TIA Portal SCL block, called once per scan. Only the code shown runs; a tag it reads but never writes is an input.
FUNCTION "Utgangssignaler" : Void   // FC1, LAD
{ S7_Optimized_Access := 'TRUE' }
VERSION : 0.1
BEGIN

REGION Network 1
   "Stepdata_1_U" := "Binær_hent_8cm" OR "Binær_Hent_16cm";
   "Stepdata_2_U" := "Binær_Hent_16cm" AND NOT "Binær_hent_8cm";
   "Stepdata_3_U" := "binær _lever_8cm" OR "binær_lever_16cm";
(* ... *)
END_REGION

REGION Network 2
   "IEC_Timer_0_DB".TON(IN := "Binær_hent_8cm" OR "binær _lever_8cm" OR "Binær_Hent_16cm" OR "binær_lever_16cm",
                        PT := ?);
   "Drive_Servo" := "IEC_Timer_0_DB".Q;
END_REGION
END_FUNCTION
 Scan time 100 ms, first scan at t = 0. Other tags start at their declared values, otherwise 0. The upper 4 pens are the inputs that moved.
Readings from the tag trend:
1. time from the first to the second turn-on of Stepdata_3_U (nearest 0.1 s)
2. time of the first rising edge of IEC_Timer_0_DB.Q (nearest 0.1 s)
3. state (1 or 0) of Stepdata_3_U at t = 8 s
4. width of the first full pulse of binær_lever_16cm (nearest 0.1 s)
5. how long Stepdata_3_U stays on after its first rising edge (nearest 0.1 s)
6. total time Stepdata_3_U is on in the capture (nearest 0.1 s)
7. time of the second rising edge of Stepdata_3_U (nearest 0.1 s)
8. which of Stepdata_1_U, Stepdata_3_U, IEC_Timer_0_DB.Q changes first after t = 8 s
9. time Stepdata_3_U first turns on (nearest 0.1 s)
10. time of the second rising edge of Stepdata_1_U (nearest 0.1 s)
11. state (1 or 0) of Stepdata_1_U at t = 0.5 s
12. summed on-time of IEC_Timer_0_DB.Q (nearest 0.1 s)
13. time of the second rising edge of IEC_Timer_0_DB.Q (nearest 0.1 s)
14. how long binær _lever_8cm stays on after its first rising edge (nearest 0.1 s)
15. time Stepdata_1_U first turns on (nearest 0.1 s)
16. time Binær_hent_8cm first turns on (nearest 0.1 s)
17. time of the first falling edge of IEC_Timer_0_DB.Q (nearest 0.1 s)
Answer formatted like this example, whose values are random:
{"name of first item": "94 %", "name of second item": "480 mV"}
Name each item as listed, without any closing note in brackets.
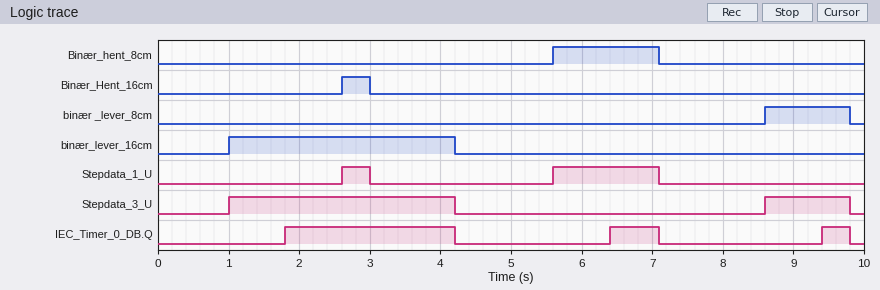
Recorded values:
{"time from the first to the second turn-on of Stepdata_3_U": "7.6 s", "time of the first rising edge of IEC_Timer_0_DB.Q": "1.8 s", "state (1 or 0) of Stepdata_3_U at t = 8 s": "0", "width of the first full pulse of binær_lever_16cm": "3.2 s", "how long Stepdata_3_U stays on after its first rising edge": "3.2 s", "total time Stepdata_3_U is on in the capture": "4.4 s", "time of the second rising edge of Stepdata_3_U": "8.6 s", "which of Stepdata_1_U, Stepdata_3_U, IEC_Timer_0_DB.Q changes first after t = 8 s": "Stepdata_3_U", "time Stepdata_3_U first turns on": "1.0 s", "time of the second rising edge of Stepdata_1_U": "5.6 s", "state (1 or 0) of Stepdata_1_U at t = 0.5 s": "0", "summed on-time of IEC_Timer_0_DB.Q": "3.5 s", "time of the second rising edge of IEC_Timer_0_DB.Q": "6.4 s", "how long binær _lever_8cm stays on after its first rising edge": "1.2 s", "time Stepdata_1_U first turns on": "2.6 s", "time Binær_hent_8cm first turns on": "5.6 s", "time of the first falling edge of IEC_Timer_0_DB.Q": "4.2 s"}
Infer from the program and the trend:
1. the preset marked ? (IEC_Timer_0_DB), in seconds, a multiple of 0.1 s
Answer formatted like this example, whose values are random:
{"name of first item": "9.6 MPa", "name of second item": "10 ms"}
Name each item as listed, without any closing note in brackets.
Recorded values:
{"the preset marked ? (IEC_Timer_0_DB), in seconds, a multiple of 0.1 s": "0.8 s"}
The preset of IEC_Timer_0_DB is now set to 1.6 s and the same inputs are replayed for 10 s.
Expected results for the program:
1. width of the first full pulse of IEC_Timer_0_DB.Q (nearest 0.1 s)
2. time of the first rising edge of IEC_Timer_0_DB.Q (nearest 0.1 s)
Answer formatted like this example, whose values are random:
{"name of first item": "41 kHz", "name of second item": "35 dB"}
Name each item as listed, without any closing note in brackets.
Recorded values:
{"width of the first full pulse of IEC_Timer_0_DB.Q": "1.6 s", "time of the first rising edge of IEC_Timer_0_DB.Q": "2.6 s"}
